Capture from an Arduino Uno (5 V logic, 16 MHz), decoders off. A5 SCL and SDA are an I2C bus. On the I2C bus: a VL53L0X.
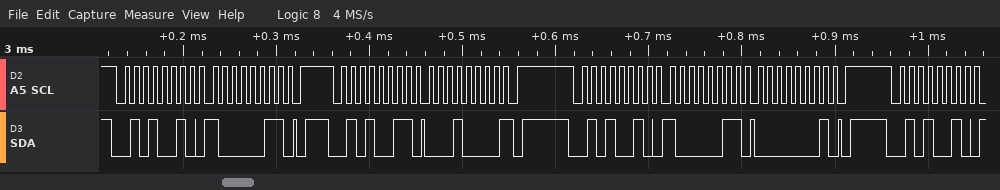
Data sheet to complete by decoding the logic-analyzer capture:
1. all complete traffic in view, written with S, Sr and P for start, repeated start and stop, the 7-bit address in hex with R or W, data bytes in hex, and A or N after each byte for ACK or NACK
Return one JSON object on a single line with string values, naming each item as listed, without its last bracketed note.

{"all complete traffic in view, written with S, Sr and P for start, repeated start and stop, the 7-bit address in hex with R or W, data bytes in hex, and A or N after each byte for ACK or NACK": "S 29W A 83 A P S 29R A 10 N P S 29W A 83 A 01 A P S 29W A"}
